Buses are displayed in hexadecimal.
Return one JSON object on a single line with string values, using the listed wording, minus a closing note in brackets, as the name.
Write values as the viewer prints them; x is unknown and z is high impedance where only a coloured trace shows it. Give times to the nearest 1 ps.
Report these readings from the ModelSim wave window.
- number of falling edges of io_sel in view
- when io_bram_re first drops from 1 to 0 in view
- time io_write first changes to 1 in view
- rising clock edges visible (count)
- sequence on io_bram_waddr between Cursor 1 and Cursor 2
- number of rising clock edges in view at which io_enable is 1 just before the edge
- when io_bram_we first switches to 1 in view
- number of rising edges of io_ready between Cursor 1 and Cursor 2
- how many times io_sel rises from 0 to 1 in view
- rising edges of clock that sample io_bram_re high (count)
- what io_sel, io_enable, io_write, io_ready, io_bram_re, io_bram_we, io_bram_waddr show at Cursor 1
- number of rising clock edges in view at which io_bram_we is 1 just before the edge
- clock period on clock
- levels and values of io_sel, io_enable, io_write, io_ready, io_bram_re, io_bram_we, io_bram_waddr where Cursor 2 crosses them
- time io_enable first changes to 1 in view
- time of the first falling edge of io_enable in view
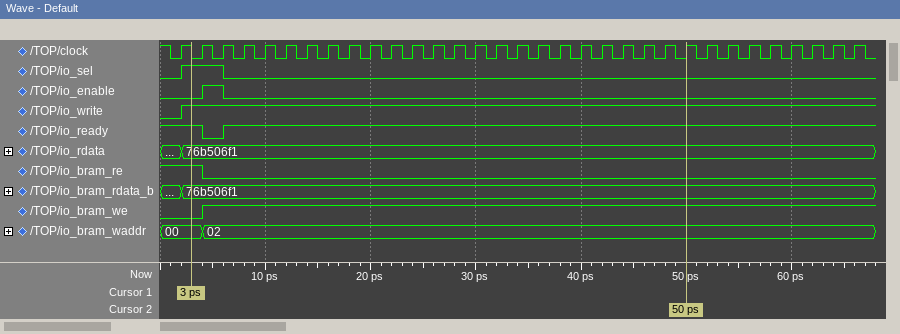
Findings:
{"number of falling edges of io_sel in view": "1", "when io_bram_re first drops from 1 to 0 in view": "4 ps", "time io_write first changes to 1 in view": "2 ps", "rising clock edges visible": "33", "sequence on io_bram_waddr between Cursor 1 and Cursor 2": "00, 02", "number of rising clock edges in view at which io_enable is 1 just before the edge": "1", "when io_bram_we first switches to 1 in view": "4 ps", "number of rising edges of io_ready between Cursor 1 and Cursor 2": "1", "how many times io_sel rises from 0 to 1 in view": "1", "rising edges of clock that sample io_bram_re high": "2", "what io_sel, io_enable, io_write, io_ready, io_bram_re, io_bram_we, io_bram_waddr show at Cursor 1": "io_sel=1, io_enable=0, io_write=1, io_ready=1, io_bram_re=1, io_bram_we=0, io_bram_waddr=00", "number of rising clock edges in view at which io_bram_we is 1 just before the edge": "31", "clock period on clock": "2 ps", "levels and values of io_sel, io_enable, io_write, io_ready, io_bram_re, io_bram_we, io_bram_waddr where Cursor 2 crosses them": "io_sel=0, io_enable=0, io_write=1, io_ready=1, io_bram_re=0, io_bram_we=1, io_bram_waddr=02", "time io_enable first changes to 1 in view": "4 ps", "time of the first falling edge of io_enable in view": "6 ps"}
